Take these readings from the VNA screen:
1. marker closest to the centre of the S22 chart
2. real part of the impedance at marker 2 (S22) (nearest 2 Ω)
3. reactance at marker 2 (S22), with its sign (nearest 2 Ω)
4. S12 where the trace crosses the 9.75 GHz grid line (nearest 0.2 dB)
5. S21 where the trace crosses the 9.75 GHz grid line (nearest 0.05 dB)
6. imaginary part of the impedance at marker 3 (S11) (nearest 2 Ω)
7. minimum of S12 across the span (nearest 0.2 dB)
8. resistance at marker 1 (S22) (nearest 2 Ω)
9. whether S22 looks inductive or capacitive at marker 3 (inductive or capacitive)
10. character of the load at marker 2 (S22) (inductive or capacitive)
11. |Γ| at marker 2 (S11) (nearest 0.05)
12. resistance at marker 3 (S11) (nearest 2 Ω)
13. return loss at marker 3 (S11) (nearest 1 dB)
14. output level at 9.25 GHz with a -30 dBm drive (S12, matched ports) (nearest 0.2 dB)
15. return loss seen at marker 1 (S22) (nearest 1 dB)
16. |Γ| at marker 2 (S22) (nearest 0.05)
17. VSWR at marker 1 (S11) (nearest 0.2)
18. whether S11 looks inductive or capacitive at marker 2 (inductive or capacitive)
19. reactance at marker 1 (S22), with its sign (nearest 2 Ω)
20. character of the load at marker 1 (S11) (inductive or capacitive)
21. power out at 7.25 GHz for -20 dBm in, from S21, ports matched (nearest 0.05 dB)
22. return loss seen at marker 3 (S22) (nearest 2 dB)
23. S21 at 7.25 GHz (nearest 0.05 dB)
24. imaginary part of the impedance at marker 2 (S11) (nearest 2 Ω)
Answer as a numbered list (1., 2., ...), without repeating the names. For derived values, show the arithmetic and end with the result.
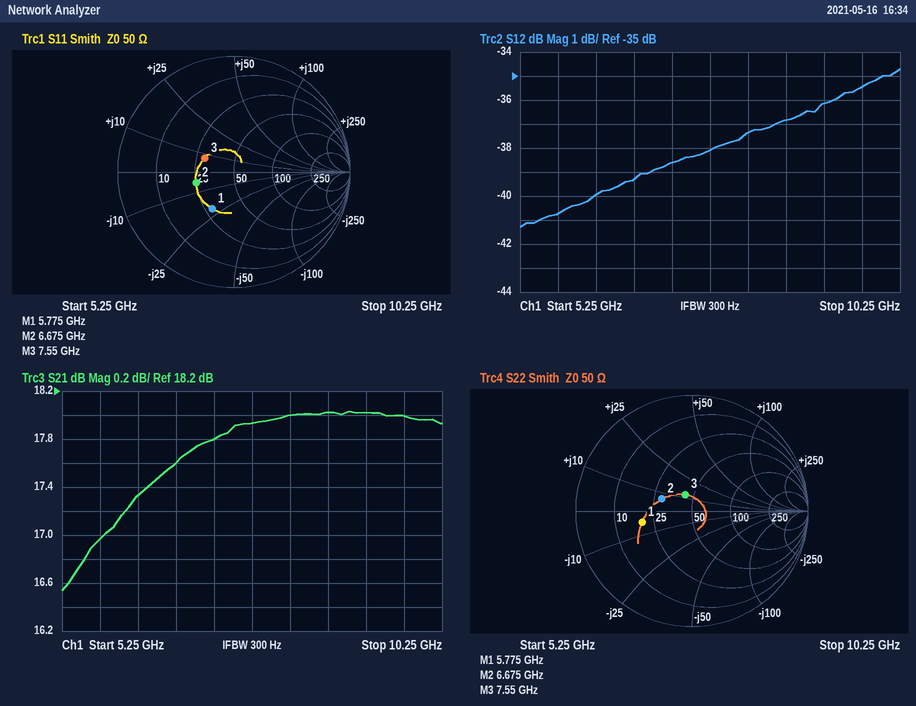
1. marker 3
2. 28 Ω
3. +6 Ω
4. -35.4 dB
5. 18.00 dB
6. +8 Ω
7. -41.2 dB
8. 20 Ω
9. inductive
10. inductive
11. 0.35
12. 30 Ω
13. 11 dB
14. -30 dBm + (-36.2 dB) = -66.2 dBm
15. 7 dB
16. 0.30
17. 2.2
18. capacitive
19. -4 Ω
20. capacitive
21. -20 dBm + (17.80 dB) = -2.20 dBm
22. 16 dB
23. 17.80 dB
24. -6 Ω
